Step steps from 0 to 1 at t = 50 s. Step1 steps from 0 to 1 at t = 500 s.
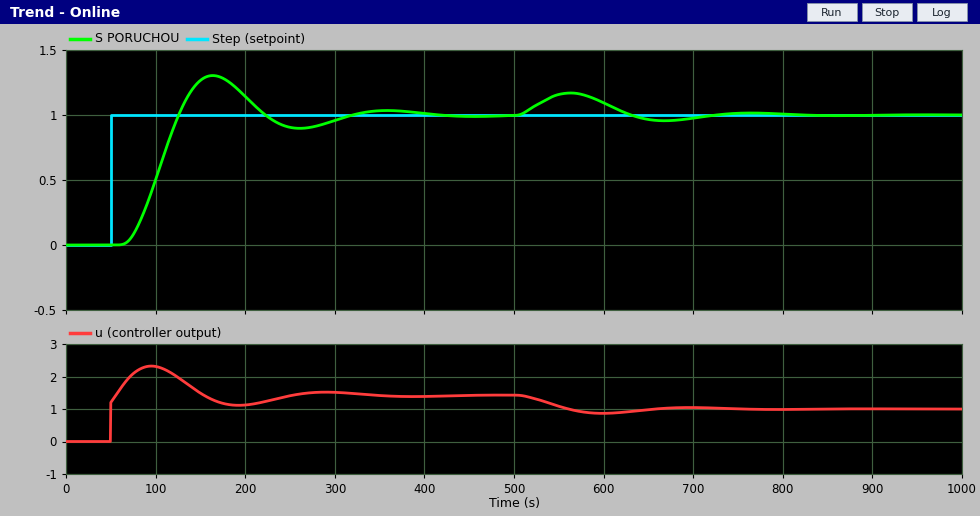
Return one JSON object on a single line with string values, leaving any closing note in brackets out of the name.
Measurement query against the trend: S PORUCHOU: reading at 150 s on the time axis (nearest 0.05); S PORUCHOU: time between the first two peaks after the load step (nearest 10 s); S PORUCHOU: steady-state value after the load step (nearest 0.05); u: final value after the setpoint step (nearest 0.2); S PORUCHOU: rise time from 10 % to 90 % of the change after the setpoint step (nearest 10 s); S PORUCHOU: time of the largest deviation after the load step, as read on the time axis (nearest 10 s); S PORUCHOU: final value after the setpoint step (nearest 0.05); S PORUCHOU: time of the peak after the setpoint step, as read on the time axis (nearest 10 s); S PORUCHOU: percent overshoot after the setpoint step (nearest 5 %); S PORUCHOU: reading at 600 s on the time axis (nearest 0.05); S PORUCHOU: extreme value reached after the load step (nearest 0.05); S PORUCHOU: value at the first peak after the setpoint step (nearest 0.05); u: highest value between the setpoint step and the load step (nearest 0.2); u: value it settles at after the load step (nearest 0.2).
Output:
{"S PORUCHOU: reading at 150 s on the time axis": "1.25", "S PORUCHOU: time between the first two peaks after the load step": "200 s", "S PORUCHOU: steady-state value after the load step": "1.00", "u: final value after the setpoint step": "1.4", "S PORUCHOU: rise time from 10 % to 90 % of the change after the setpoint step": "40 s", "S PORUCHOU: time of the largest deviation after the load step, as read on the time axis": "560 s", "S PORUCHOU: final value after the setpoint step": "1.00", "S PORUCHOU: time of the peak after the setpoint step, as read on the time axis": "160 s", "S PORUCHOU: percent overshoot after the setpoint step": "30 %", "S PORUCHOU: reading at 600 s on the time axis": "1.10", "S PORUCHOU: extreme value reached after the load step": "1.15", "S PORUCHOU: value at the first peak after the setpoint step": "1.30", "u: highest value between the setpoint step and the load step": "2.4", "u: value it settles at after the load step": "1.0"}
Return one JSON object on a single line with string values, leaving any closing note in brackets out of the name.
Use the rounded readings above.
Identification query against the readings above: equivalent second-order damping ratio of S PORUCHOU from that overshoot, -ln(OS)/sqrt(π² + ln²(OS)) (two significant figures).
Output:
{"equivalent second-order damping ratio of S PORUCHOU from that overshoot, -ln(OS)/sqrt(π² + ln²(OS))": "0.36"}
